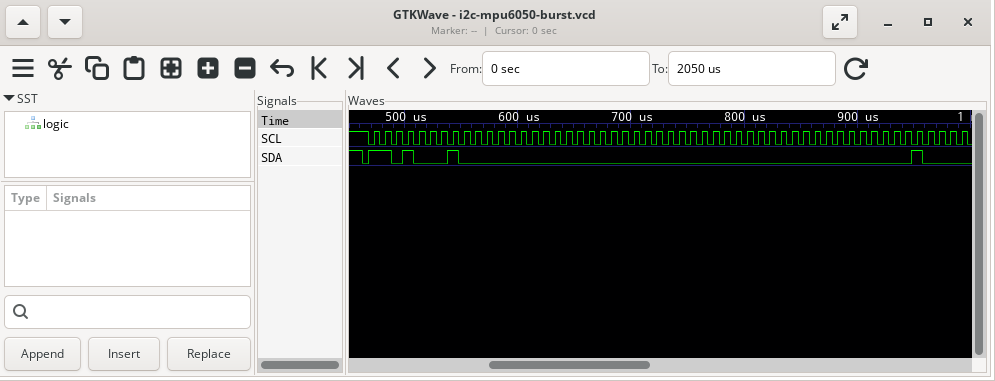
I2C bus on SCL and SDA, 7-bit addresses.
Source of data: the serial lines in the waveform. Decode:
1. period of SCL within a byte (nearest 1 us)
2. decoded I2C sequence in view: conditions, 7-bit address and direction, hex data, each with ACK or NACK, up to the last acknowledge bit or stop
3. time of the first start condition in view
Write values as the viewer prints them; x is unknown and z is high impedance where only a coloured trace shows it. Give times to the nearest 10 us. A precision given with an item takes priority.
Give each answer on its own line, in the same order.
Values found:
10 us
start, address 68 read ACK, 00 ACK, 00 ACK, 00 ACK, 00 ACK
460 us
